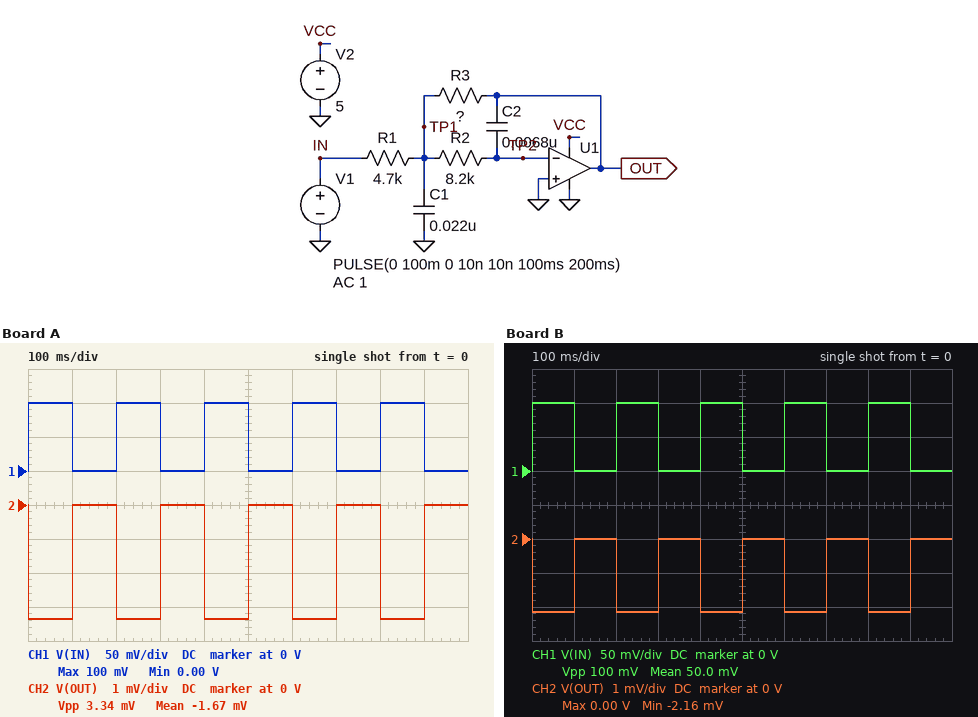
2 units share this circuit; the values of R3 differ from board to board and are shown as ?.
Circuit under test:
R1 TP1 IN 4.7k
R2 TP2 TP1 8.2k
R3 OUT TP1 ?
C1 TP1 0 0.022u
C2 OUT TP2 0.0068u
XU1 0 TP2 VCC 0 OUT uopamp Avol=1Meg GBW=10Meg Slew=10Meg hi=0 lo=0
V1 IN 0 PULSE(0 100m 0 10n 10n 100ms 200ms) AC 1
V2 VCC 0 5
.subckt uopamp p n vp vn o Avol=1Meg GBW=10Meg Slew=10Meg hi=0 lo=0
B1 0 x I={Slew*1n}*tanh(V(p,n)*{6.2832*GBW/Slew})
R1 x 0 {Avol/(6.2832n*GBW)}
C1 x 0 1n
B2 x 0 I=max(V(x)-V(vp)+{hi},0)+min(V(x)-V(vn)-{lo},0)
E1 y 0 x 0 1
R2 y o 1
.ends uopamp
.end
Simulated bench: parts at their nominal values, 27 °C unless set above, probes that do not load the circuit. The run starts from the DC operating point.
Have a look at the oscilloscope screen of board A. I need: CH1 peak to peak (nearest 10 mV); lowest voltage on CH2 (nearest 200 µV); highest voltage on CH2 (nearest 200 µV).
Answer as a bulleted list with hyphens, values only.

- 100 mV
- -3.4 mV
- 0 V
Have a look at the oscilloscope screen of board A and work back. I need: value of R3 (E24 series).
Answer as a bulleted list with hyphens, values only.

- 6.2 kΩ
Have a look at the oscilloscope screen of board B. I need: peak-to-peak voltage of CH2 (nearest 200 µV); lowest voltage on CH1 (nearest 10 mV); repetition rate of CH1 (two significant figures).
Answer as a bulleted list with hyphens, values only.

- 2.2 mV
- 0 V
- 5.0 Hz
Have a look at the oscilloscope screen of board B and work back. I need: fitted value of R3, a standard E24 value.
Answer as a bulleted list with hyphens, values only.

- 2.7 kΩ
